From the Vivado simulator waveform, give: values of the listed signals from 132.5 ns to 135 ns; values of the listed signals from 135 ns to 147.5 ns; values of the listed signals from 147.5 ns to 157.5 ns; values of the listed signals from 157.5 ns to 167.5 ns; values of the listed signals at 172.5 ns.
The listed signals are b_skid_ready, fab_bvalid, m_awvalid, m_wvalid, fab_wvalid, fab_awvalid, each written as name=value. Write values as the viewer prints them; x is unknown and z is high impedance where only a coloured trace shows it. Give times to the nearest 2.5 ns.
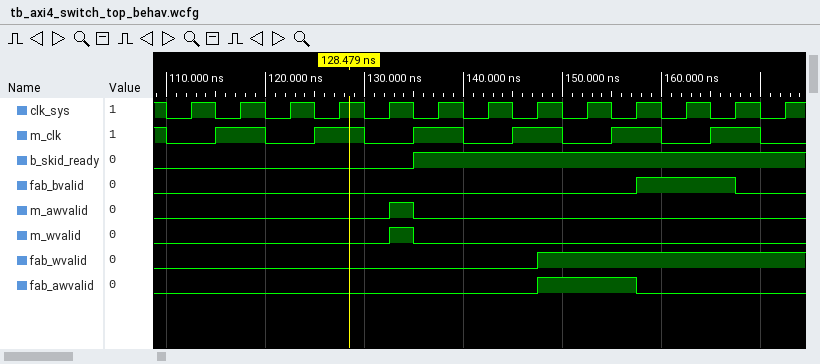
b_skid_ready=0, fab_bvalid=0, m_awvalid=1, m_wvalid=1, fab_wvalid=0, fab_awvalid=0
b_skid_ready=1, fab_bvalid=0, m_awvalid=0, m_wvalid=0, fab_wvalid=0, fab_awvalid=0
b_skid_ready=1, fab_bvalid=0, m_awvalid=0, m_wvalid=0, fab_wvalid=1, fab_awvalid=1
b_skid_ready=1, fab_bvalid=1, m_awvalid=0, m_wvalid=0, fab_wvalid=1, fab_awvalid=0
b_skid_ready=1, fab_bvalid=0, m_awvalid=0, m_wvalid=0, fab_wvalid=1, fab_awvalid=0
